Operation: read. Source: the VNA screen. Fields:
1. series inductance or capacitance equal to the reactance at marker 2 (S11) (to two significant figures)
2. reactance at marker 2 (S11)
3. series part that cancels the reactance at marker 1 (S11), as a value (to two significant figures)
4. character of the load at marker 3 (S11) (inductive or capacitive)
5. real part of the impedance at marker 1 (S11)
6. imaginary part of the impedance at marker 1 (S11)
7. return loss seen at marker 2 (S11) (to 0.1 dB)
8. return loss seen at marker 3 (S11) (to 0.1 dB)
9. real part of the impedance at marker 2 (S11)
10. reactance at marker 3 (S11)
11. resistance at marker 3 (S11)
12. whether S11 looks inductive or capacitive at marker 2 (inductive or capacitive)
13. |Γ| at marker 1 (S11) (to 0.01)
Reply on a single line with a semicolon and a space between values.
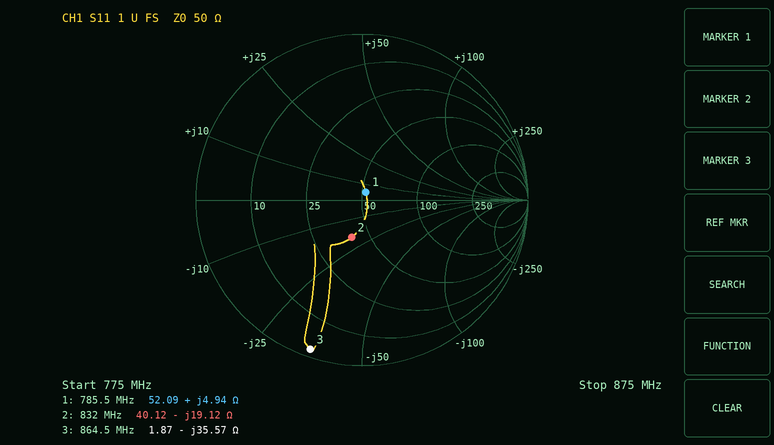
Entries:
10 pF; -19.12 Ω; 41 pF; capacitive; 52.09 Ω; +4.94 Ω; 12.6 dB; 0.4 dB; 40.12 Ω; -35.57 Ω; 1.87 Ω; capacitive; 0.05
